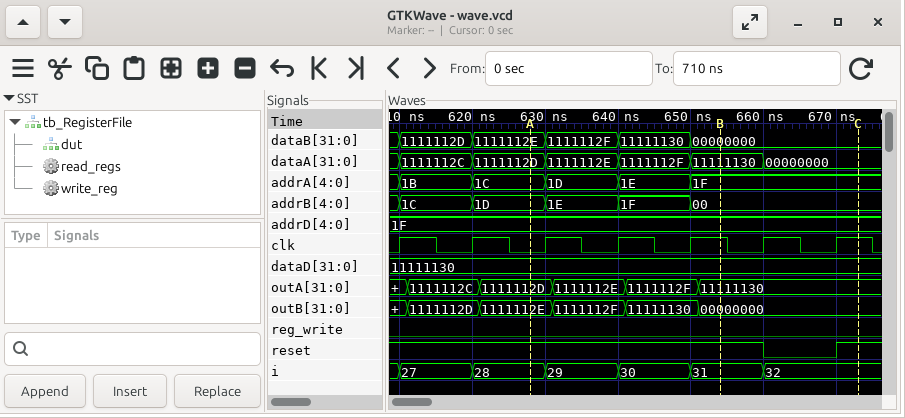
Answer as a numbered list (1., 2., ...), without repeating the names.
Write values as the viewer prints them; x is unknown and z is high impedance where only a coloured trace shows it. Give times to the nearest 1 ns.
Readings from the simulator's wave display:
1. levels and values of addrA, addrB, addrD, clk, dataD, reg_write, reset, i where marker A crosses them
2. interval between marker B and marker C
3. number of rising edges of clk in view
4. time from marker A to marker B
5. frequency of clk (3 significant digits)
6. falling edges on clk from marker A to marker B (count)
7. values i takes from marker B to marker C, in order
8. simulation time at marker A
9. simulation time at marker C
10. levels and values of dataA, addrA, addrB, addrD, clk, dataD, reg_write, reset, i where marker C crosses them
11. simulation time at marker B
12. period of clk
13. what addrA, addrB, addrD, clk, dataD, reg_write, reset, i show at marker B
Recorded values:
1. addrA=1C, addrB=1D, addrD=1F, clk=0, dataD=11111130, reg_write=0, reset=1, i=28
2. 19 ns
3. 7
4. 26 ns
5. 100 MHz
6. 2
7. 31, 32
8. 628 ns
9. 673 ns
10. dataA=00000000, addrA=1F, addrB=00, addrD=1F, clk=1, dataD=11111130, reg_write=0, reset=1, i=32
11. 654 ns
12. 10 ns
13. addrA=1F, addrB=00, addrD=1F, clk=1, dataD=11111130, reg_write=0, reset=1, i=31
